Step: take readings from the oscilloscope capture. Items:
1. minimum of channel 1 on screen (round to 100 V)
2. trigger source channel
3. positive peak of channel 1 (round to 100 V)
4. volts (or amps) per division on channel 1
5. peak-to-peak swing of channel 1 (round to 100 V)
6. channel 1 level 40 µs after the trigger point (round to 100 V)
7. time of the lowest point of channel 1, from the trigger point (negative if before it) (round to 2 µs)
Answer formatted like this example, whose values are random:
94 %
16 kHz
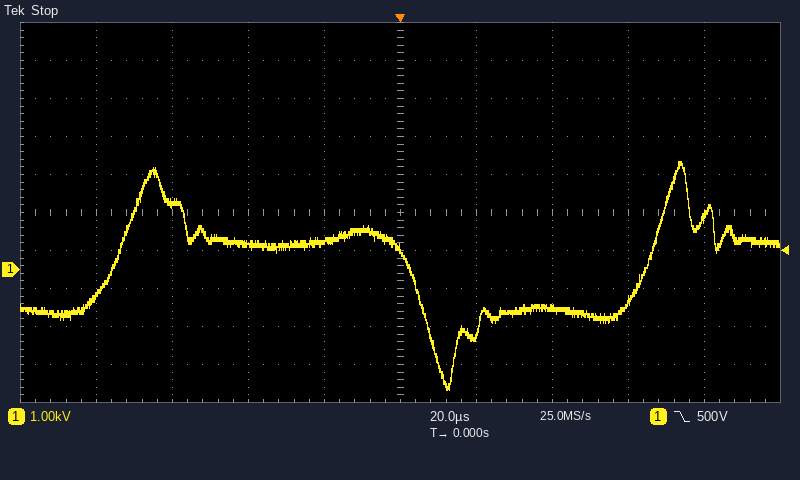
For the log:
-3.2 kV
channel 1
2.8 kV
1 kV
6.0 kV
-1.0 kV
+12 µs
